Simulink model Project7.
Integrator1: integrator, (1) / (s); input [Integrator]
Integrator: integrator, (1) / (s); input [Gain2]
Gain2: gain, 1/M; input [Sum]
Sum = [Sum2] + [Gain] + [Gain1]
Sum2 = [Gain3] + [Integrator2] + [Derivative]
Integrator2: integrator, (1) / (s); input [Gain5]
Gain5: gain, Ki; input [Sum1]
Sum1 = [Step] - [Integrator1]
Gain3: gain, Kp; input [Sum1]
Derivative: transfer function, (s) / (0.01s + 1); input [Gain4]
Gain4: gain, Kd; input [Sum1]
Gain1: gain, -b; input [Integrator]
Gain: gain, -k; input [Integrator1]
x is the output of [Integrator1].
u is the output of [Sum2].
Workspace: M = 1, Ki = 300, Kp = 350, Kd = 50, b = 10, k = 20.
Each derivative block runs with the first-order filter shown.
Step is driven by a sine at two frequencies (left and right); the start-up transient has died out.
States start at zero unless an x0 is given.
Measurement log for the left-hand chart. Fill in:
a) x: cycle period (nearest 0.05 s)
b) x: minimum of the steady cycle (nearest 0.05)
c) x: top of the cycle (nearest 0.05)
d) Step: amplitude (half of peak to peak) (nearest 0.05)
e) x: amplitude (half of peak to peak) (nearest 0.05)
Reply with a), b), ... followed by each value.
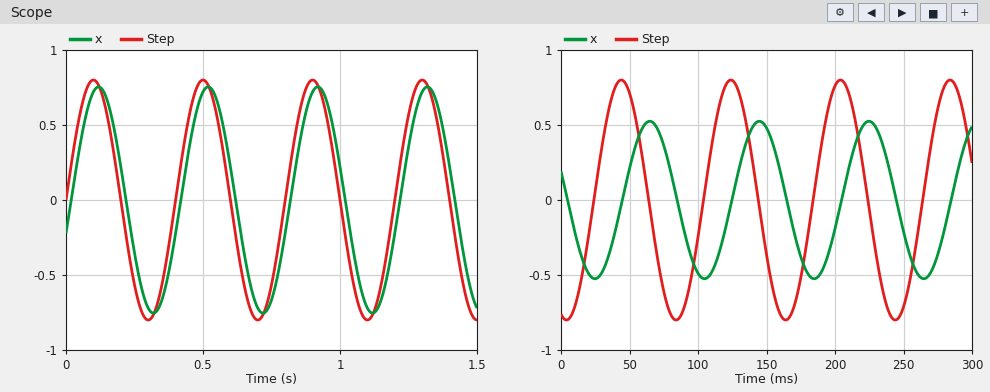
a) 0.40 s
b) -0.75
c) 0.75
d) 0.80
e) 0.75
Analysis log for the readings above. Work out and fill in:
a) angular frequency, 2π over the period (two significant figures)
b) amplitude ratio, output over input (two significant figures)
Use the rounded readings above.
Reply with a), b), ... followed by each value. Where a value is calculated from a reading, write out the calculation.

a) 2π / 0.4 = 16 rad/s
b) 0.75 / 0.8 = 0.94
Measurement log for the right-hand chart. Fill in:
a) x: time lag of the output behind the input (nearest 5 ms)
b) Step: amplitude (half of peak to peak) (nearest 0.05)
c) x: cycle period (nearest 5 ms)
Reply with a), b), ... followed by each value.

a) 20 ms
b) 0.80
c) 80 ms
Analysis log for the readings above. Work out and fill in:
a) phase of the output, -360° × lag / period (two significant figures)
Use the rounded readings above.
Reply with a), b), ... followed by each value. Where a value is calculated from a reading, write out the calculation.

a) -360 × 20 / 80 = -90°
